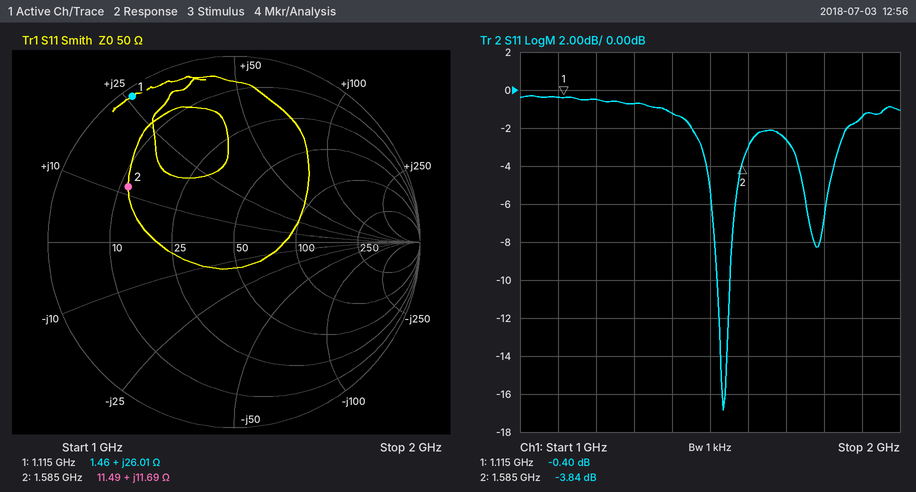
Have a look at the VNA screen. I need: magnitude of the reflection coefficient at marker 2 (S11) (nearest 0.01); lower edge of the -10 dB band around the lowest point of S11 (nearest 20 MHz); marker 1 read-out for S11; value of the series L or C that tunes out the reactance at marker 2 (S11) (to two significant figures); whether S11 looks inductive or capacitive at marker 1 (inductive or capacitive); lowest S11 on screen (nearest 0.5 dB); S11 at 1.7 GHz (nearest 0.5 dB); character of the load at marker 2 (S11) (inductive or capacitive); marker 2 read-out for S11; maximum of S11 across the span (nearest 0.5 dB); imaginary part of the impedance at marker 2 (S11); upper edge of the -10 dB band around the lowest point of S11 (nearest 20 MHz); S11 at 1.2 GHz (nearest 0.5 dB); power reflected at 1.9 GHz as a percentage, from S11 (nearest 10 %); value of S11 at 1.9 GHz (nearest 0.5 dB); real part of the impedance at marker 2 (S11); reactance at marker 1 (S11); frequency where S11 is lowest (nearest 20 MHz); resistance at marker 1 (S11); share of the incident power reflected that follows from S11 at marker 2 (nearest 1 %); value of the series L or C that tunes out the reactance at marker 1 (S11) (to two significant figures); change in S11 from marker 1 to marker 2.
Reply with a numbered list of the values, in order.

1. 0.64
2. 1.52 GHz
3. -0.40 dB
4. 8.6 pF
5. inductive
6. -17.0 dB
7. -2.5 dB
8. inductive
9. -3.84 dB
10. -0.5 dB
11. +11.69 Ω
12. 1.56 GHz
13. -0.5 dB
14. 70 %
15. -1.5 dB
16. 11.49 Ω
17. +26.01 Ω
18. 1.54 GHz
19. 1.46 Ω
20. 41 %
21. 5.5 pF
22. -3.44 dB
